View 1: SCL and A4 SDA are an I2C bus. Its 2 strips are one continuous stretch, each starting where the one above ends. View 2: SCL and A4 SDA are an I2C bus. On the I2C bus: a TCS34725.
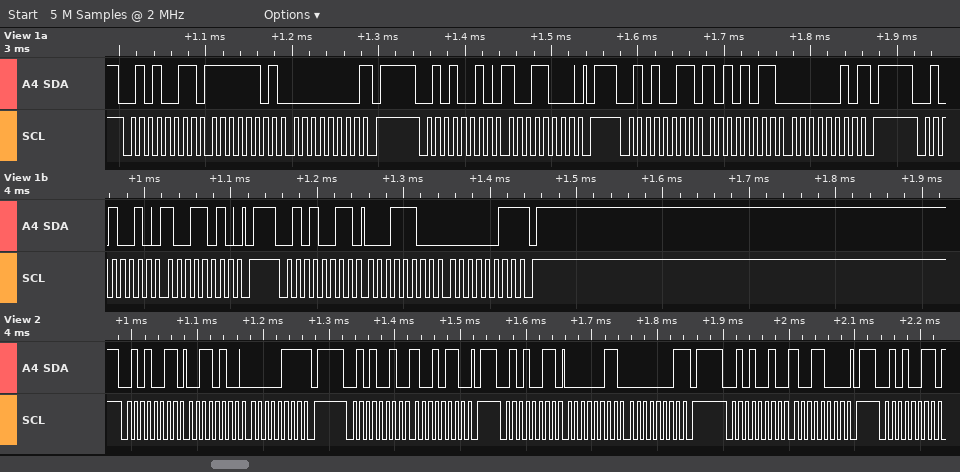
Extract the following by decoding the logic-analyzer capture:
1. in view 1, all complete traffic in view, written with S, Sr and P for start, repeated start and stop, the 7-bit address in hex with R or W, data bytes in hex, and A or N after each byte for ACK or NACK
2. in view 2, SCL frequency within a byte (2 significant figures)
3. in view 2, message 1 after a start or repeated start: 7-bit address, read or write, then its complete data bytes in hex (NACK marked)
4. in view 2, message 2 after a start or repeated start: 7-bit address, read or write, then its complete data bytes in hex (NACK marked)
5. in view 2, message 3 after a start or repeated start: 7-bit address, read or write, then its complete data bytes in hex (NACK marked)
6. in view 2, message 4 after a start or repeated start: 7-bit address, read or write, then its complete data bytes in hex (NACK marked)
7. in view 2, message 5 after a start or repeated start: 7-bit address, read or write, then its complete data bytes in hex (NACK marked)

S 29R A FD A 00 N P S 29W A 98 A P S 29R A AB A 02 N P S 29W A 9A A P S 29R A 1C A 03 N P
100 kHz
0x29 read: 34 07 NACK
0x29 write: 96
0x29 read: 03 01 NACK
0x29 write: 98
0x29 read
